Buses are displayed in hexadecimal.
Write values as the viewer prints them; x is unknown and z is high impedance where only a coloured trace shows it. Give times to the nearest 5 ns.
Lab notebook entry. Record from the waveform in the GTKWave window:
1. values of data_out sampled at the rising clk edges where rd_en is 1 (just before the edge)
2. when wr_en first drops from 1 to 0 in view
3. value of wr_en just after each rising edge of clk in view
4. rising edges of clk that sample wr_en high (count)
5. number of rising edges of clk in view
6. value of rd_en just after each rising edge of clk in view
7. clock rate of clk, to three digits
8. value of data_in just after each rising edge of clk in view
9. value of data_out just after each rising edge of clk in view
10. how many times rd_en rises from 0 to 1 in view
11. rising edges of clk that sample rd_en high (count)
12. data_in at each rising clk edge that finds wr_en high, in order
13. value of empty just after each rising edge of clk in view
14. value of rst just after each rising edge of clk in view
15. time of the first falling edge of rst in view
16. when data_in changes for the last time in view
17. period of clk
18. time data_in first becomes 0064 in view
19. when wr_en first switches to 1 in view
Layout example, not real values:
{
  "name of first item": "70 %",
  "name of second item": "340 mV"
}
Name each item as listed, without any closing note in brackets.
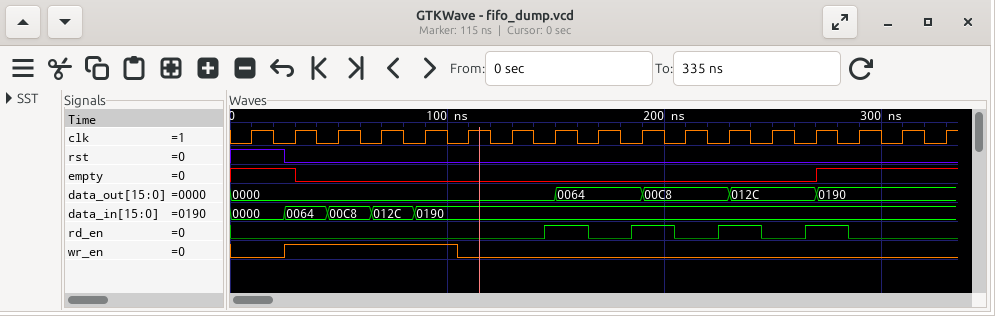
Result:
{
  "values of data_out sampled at the rising clk edges where rd_en is 1": "0000, 0064, 00C8, 012C",
  "when wr_en first drops from 1 to 0 in view": "105 ns",
  "value of wr_en just after each rising edge of clk in view": "0 1 1 1 1 0 0 0 0 0 0 0 0 0 0 0 0",
  "rising edges of clk that sample wr_en high": "4",
  "number of rising edges of clk in view": "17",
  "value of rd_en just after each rising edge of clk in view": "0 0 0 0 0 0 0 1 0 1 0 1 0 1 0 0 0",
  "clock rate of clk, to three digits": "50.0 MHz",
  "value of data_in just after each rising edge of clk in view": "0000, 0064, 00C8, 012C, 0190, 0190, 0190, 0190, 0190, 0190, 0190, 0190, 0190, 0190, 0190, 0190, 0190",
  "value of data_out just after each rising edge of clk in view": "0000, 0000, 0000, 0000, 0000, 0000, 0000, 0064, 0064, 00C8, 00C8, 012C, 012C, 0190, 0190, 0190, 0190",
  "how many times rd_en rises from 0 to 1 in view": "4",
  "rising edges of clk that sample rd_en high": "4",
  "data_in at each rising clk edge that finds wr_en high, in order": "0064, 00C8, 012C, 0190",
  "value of empty just after each rising edge of clk in view": "1 0 0 0 0 0 0 0 0 0 0 0 0 1 1 1 1",
  "value of rst just after each rising edge of clk in view": "1 0 0 0 0 0 0 0 0 0 0 0 0 0 0 0 0",
  "time of the first falling edge of rst in view": "25 ns",
  "when data_in changes for the last time in view": "85 ns",
  "period of clk": "20 ns",
  "time data_in first becomes 0064 in view": "25 ns",
  "when wr_en first switches to 1 in view": "25 ns"
}
